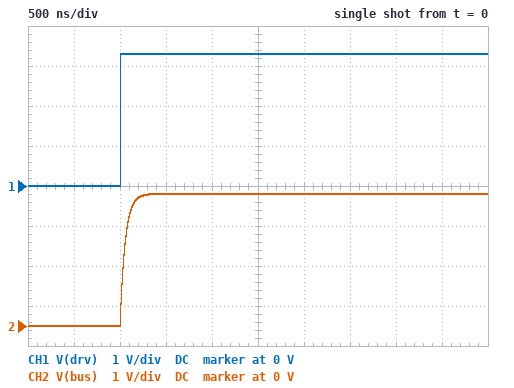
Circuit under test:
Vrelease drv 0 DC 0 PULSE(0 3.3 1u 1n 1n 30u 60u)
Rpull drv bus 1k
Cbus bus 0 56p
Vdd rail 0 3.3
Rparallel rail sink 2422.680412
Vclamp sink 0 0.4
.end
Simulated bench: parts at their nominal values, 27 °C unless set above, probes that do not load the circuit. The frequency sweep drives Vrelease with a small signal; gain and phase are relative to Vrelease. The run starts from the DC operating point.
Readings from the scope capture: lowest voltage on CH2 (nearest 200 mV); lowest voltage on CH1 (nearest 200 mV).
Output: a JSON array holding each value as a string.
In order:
["0 V", "0 V"]
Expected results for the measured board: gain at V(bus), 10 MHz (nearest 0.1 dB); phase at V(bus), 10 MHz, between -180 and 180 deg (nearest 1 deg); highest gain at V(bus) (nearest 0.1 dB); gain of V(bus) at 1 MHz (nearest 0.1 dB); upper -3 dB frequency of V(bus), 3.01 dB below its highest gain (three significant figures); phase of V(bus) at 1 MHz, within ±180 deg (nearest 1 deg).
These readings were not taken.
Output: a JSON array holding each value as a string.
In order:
["-11.3 dB", "-74 deg", "0 dB", "-0.5 dB", "2.84 MHz", "-19 deg"]
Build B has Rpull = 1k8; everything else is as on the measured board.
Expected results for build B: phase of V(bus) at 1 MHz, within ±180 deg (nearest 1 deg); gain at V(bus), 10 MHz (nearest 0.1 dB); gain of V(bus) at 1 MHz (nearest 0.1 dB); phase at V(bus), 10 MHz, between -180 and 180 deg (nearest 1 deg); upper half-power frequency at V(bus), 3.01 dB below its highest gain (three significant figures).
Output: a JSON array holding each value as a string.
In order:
["-32 deg", "-16.1 dB", "-1.5 dB", "-81 deg", "1.58 MHz"]
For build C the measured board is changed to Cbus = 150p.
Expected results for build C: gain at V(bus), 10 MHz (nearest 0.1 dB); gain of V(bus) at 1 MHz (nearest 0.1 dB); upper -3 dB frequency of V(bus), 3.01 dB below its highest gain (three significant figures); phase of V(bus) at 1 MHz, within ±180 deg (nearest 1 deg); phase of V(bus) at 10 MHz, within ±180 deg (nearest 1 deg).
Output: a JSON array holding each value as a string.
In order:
["-19.5 dB", "-2.8 dB", "1.06 MHz", "-43 deg", "-84 deg"]
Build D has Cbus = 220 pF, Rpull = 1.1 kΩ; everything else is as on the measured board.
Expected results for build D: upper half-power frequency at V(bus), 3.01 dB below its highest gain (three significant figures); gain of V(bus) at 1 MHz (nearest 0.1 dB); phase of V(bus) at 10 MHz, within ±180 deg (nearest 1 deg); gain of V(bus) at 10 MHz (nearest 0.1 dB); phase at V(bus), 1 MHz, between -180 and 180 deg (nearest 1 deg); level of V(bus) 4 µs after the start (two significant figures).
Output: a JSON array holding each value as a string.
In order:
["658 kHz", "-5.2 dB", "-86 deg", "-23.7 dB", "-57 deg", "3.3 V"]
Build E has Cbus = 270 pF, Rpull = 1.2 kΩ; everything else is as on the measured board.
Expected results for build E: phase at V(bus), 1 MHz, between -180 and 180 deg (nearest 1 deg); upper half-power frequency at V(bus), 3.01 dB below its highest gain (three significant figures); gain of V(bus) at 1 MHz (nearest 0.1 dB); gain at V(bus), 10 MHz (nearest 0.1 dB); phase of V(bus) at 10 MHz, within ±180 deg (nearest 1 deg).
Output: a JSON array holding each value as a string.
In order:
["-64 deg", "491 kHz", "-7.1 dB", "-26.2 dB", "-87 deg"]
